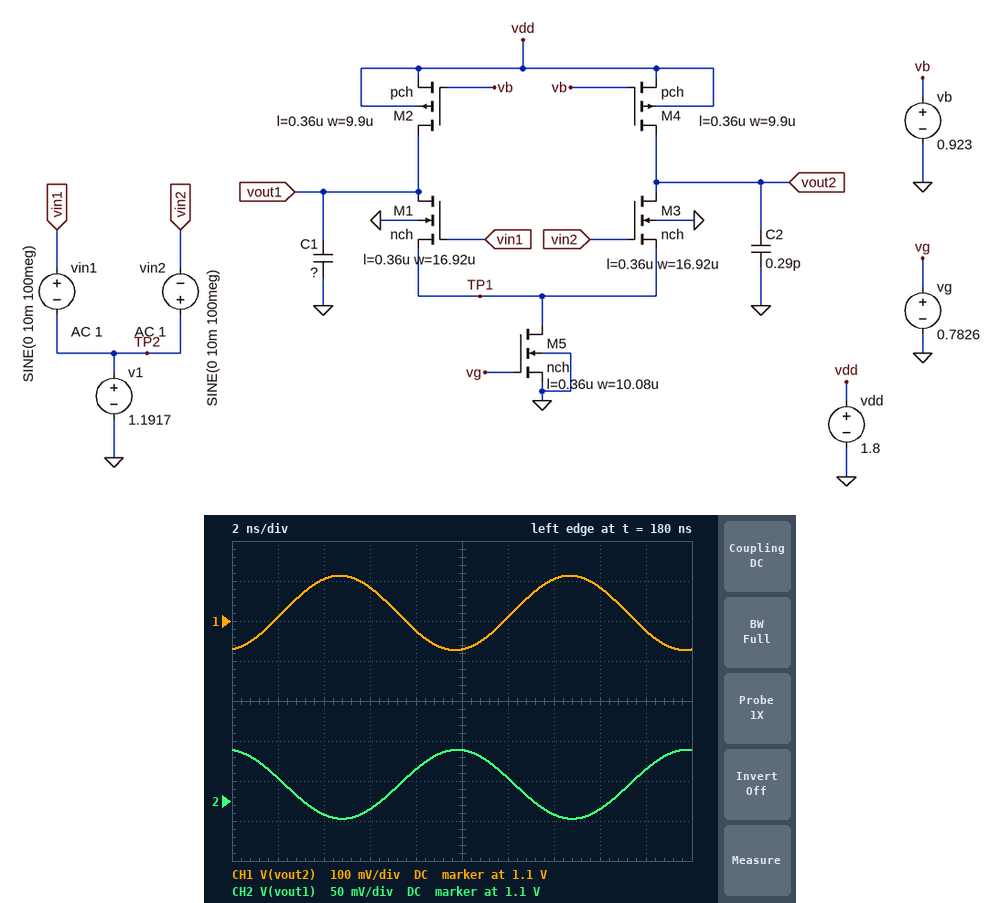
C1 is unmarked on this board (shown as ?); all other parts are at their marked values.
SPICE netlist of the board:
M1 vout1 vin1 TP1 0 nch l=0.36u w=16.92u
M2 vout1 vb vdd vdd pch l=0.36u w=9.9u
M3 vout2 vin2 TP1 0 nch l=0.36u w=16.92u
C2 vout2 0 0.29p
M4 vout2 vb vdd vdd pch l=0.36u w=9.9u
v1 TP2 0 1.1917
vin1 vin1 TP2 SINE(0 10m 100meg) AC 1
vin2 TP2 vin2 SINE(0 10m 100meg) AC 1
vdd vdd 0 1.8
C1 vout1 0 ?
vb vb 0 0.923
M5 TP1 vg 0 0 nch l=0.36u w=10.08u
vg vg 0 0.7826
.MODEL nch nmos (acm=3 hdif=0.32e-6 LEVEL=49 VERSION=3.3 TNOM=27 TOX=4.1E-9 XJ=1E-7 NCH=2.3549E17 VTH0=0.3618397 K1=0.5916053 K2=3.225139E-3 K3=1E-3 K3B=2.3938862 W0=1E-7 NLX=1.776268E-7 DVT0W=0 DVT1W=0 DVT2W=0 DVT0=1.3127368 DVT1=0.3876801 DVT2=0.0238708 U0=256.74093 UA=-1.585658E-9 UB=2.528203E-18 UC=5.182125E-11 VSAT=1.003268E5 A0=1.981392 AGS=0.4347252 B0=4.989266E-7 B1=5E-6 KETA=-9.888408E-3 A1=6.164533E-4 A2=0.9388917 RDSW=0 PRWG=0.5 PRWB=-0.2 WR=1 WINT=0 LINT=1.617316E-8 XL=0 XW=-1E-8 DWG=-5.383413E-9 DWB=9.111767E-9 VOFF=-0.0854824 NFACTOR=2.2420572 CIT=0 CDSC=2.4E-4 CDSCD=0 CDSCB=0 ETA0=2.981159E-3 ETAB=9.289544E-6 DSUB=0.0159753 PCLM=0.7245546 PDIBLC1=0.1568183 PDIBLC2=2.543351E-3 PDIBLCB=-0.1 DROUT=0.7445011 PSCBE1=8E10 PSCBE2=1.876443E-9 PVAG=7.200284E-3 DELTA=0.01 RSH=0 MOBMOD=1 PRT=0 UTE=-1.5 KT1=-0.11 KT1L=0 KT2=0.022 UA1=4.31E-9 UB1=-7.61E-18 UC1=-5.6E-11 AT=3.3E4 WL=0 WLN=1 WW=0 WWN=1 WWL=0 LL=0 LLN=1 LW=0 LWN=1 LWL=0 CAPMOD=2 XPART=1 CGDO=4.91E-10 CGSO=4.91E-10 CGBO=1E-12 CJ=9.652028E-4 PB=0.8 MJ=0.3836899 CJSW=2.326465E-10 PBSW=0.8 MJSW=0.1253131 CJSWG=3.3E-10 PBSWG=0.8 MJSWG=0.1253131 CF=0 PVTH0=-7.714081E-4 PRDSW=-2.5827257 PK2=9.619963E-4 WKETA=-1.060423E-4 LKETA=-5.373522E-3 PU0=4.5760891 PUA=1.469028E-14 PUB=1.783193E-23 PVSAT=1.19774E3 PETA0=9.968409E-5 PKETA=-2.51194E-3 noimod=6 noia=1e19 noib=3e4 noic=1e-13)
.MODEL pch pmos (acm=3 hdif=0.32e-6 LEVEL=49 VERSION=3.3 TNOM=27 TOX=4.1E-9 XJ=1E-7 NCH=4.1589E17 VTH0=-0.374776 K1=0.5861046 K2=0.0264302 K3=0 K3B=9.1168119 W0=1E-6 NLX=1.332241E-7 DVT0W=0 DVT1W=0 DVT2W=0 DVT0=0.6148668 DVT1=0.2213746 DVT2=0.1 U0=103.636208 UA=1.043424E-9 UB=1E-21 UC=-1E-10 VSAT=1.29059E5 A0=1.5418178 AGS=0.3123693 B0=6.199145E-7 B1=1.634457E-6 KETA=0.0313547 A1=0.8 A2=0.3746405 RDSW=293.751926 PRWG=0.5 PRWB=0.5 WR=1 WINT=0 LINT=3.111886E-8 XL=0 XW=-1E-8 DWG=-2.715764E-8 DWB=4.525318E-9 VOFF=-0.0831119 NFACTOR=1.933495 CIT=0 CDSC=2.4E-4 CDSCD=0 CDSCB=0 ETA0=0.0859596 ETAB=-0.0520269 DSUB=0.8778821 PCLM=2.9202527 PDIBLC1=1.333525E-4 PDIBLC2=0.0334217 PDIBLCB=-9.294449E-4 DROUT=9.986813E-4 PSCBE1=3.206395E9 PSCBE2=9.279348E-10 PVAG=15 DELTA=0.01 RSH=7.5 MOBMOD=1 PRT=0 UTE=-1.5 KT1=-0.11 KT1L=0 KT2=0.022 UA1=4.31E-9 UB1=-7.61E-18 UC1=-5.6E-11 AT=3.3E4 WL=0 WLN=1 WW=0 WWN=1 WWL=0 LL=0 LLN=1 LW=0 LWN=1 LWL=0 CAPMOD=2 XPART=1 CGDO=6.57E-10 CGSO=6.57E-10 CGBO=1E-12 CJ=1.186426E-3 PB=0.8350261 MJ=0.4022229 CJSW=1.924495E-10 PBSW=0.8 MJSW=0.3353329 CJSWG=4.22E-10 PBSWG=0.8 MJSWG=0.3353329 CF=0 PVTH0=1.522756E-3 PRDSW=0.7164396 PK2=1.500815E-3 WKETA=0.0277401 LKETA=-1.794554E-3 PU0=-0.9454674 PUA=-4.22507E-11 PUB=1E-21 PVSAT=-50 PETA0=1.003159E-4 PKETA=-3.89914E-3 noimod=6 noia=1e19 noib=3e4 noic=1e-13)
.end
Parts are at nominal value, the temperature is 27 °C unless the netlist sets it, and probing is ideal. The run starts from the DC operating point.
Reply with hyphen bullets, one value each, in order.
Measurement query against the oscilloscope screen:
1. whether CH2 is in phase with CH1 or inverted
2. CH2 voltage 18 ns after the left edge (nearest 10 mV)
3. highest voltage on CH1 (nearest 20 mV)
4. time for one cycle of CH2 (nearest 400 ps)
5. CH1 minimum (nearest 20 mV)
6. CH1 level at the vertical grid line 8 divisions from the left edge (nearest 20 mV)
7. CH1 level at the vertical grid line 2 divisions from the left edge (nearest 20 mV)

- inverted
- 1.14 V
- 1.22 V
- 10.0 ns
- 1.02 V
- 1.18 V
- 1.20 V
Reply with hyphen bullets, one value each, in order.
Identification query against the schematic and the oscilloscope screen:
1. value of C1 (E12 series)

- 680 fF
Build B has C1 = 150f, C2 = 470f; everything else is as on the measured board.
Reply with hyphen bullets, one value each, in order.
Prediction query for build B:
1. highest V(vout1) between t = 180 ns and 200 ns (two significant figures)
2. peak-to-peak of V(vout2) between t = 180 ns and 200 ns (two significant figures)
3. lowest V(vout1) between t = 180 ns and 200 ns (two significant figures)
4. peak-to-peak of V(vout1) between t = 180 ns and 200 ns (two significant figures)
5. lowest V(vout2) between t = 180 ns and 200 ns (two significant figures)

- 1.3 V
- 120 mV
- 960 mV
- 310 mV
- 1.1 V
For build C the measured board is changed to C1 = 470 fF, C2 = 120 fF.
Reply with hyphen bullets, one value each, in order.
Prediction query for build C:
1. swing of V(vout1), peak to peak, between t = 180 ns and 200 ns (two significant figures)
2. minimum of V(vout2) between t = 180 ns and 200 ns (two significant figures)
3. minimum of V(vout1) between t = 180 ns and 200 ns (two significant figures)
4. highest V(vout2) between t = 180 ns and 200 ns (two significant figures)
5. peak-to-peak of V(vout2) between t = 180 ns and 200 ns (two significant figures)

- 120 mV
- 930 mV
- 1.1 V
- 1.3 V
- 360 mV
